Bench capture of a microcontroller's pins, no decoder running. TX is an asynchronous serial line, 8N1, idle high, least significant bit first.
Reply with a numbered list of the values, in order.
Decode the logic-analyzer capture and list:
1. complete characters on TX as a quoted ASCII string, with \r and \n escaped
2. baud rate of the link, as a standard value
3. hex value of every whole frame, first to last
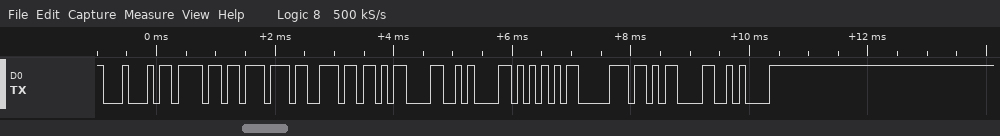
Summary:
1. "Down\r\nUp\r\n"
2. 9600 baud
3. 44 6F 77 6E 0D 0A 55 70 0D 0A
